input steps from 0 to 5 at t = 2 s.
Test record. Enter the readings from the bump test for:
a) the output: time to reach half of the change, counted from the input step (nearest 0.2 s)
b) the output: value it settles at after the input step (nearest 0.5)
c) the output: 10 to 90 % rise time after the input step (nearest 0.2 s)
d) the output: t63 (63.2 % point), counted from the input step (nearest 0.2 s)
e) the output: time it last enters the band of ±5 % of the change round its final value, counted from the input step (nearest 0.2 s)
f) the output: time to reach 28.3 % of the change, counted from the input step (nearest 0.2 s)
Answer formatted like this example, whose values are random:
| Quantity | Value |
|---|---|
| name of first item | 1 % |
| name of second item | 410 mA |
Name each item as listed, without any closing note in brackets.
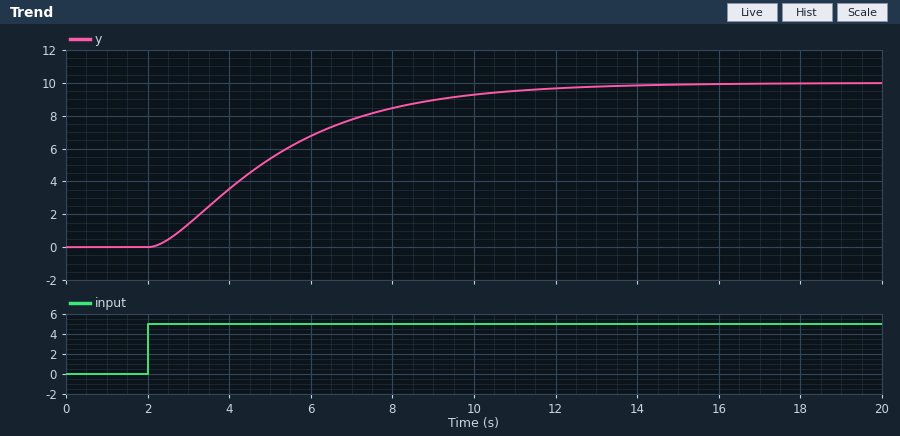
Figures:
| Quantity | Value |
|---|---|
| the output: time to reach half of the change, counted from the input step | 2.8 s |
| the output: value it settles at after the input step | 10.0 |
| the output: 10 to 90 % rise time after the input step | 6.4 s |
| the output: t63 (63.2 % point), counted from the input step | 3.6 s |
| the output: time it last enters the band of ±5 % of the change round its final value, counted from the input step | 9.0 s |
| the output: time to reach 28.3 % of the change, counted from the input step | 1.6 s |
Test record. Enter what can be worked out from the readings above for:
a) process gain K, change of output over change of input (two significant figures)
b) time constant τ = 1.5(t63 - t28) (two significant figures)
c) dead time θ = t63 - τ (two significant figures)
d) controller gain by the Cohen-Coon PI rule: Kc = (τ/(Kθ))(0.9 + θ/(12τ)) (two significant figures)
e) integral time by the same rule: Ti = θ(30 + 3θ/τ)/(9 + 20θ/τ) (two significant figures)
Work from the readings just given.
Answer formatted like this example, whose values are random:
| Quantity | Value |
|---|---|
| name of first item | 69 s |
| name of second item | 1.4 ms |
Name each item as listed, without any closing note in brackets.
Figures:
| Quantity | Value |
|---|---|
| process gain K, change of output over change of input | 2.0 |
| time constant τ = 1.5(t63 - t28) | 3.0 s |
| dead time θ = t63 - τ | 0.60 s |
| controller gain by the Cohen-Coon PI rule: Kc = (τ/(Kθ))(0.9 + θ/(12τ)) | 2.3 |
| integral time by the same rule: Ti = θ(30 + 3θ/τ)/(9 + 20θ/τ) | 1.4 s |
